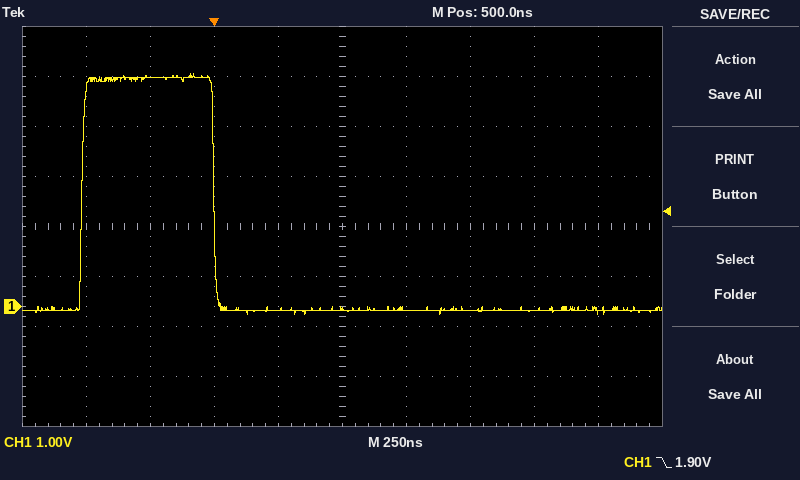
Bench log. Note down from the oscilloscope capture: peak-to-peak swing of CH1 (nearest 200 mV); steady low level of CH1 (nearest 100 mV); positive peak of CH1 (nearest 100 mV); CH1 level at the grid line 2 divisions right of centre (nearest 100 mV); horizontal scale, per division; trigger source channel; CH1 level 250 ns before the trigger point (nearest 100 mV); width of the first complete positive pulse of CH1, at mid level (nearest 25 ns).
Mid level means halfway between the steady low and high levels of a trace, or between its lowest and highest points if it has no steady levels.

4.8 V
-100 mV
4.7 V
-100 mV
250 ns
CH1
4.6 V
525 ns
